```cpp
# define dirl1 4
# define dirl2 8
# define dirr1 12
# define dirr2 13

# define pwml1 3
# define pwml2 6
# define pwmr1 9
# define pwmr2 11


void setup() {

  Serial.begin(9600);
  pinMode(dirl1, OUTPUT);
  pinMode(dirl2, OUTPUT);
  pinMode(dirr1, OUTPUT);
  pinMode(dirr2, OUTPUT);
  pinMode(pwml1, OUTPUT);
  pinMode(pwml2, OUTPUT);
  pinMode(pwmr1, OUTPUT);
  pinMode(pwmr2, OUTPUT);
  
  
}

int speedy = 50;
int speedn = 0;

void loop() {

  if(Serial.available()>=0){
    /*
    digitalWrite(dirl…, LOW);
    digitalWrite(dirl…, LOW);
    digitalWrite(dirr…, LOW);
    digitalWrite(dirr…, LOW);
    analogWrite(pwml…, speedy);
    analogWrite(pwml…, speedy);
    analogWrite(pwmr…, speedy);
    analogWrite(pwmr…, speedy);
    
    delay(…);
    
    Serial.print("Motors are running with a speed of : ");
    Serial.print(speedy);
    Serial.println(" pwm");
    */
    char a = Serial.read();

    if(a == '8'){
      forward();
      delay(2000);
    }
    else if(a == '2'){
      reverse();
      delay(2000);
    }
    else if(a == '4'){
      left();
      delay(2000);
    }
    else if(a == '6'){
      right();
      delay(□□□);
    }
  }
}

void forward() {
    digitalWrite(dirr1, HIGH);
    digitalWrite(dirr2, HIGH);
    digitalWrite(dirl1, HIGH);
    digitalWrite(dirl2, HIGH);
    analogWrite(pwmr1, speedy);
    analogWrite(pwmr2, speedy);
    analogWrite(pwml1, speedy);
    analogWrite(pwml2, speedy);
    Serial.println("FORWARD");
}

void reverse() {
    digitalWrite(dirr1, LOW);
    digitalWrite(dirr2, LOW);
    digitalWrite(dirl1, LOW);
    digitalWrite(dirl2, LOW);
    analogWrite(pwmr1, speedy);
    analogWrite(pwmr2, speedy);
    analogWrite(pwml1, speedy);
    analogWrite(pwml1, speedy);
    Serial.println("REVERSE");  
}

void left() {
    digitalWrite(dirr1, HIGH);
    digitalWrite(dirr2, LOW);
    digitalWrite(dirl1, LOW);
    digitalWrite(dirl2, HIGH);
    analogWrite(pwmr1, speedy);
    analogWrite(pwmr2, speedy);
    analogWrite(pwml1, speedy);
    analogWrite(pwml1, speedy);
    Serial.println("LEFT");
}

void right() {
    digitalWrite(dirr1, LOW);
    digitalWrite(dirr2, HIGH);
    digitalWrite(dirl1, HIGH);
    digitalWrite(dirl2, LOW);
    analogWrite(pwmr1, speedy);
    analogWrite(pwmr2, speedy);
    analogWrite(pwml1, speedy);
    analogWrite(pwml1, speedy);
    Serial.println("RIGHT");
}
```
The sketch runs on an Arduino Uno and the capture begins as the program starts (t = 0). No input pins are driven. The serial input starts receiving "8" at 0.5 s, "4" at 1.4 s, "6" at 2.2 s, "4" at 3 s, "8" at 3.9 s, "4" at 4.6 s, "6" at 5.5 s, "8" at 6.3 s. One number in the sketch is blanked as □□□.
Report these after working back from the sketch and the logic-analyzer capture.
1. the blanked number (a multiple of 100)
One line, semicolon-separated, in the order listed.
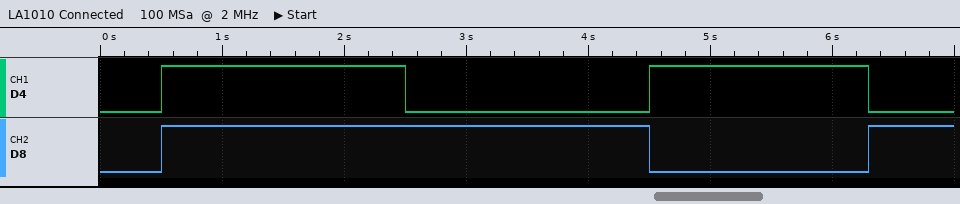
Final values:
1800
